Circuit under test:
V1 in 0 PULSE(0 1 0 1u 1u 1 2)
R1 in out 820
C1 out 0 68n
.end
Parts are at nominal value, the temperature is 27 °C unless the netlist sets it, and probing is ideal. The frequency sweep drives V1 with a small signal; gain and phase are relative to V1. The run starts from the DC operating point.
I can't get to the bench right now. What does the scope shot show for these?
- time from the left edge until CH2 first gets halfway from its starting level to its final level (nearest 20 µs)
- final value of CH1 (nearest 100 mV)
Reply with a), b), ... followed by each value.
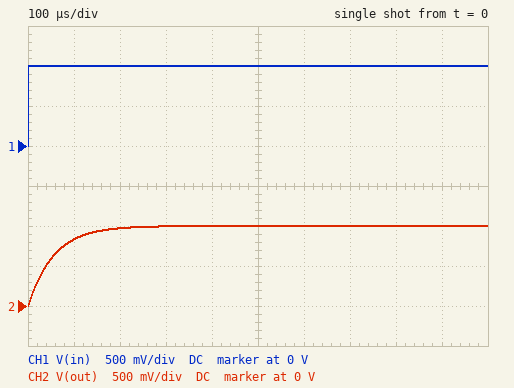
a) 40 µs
b) 1.0 V
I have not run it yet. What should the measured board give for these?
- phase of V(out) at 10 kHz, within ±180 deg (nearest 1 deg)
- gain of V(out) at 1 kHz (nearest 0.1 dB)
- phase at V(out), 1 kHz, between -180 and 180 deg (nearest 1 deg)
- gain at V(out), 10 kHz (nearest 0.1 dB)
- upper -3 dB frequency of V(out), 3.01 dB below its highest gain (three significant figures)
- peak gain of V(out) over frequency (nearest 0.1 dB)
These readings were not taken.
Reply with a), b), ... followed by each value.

a) -74 deg
b) -0.5 dB
c) -19 deg
d) -11.2 dB
e) 2.85 kHz
f) 0 dB
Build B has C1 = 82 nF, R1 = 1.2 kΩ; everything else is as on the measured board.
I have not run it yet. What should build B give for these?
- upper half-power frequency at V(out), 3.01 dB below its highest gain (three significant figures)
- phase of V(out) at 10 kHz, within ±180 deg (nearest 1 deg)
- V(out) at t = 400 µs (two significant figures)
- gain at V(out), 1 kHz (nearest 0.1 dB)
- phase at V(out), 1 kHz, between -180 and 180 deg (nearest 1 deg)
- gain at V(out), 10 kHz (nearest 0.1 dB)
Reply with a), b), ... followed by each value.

a) 1.62 kHz
b) -81 deg
c) 980 mV
d) -1.4 dB
e) -32 deg
f) -15.9 dB
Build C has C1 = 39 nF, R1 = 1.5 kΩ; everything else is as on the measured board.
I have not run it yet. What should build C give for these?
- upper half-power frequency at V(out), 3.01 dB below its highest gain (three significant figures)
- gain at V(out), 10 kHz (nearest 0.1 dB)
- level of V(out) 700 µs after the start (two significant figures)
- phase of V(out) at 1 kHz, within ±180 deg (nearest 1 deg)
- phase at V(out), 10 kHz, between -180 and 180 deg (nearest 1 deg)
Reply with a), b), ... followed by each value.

a) 2.72 kHz
b) -11.6 dB
c) 1.0 V
d) -20 deg
e) -75 deg
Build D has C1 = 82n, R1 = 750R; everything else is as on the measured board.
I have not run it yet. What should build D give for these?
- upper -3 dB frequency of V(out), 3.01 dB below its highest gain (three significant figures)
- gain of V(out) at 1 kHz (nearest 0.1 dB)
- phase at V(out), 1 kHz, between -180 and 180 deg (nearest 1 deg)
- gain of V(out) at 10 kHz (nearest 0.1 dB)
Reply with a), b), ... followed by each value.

a) 2.59 kHz
b) -0.6 dB
c) -21 deg
d) -12.0 dB
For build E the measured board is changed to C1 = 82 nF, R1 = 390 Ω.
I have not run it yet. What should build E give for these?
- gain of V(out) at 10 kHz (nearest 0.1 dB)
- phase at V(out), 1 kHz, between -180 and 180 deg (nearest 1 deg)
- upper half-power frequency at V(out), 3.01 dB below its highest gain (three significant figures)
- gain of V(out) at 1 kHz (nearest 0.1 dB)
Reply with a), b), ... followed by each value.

a) -7.0 dB
b) -11 deg
c) 4.98 kHz
d) -0.2 dB
